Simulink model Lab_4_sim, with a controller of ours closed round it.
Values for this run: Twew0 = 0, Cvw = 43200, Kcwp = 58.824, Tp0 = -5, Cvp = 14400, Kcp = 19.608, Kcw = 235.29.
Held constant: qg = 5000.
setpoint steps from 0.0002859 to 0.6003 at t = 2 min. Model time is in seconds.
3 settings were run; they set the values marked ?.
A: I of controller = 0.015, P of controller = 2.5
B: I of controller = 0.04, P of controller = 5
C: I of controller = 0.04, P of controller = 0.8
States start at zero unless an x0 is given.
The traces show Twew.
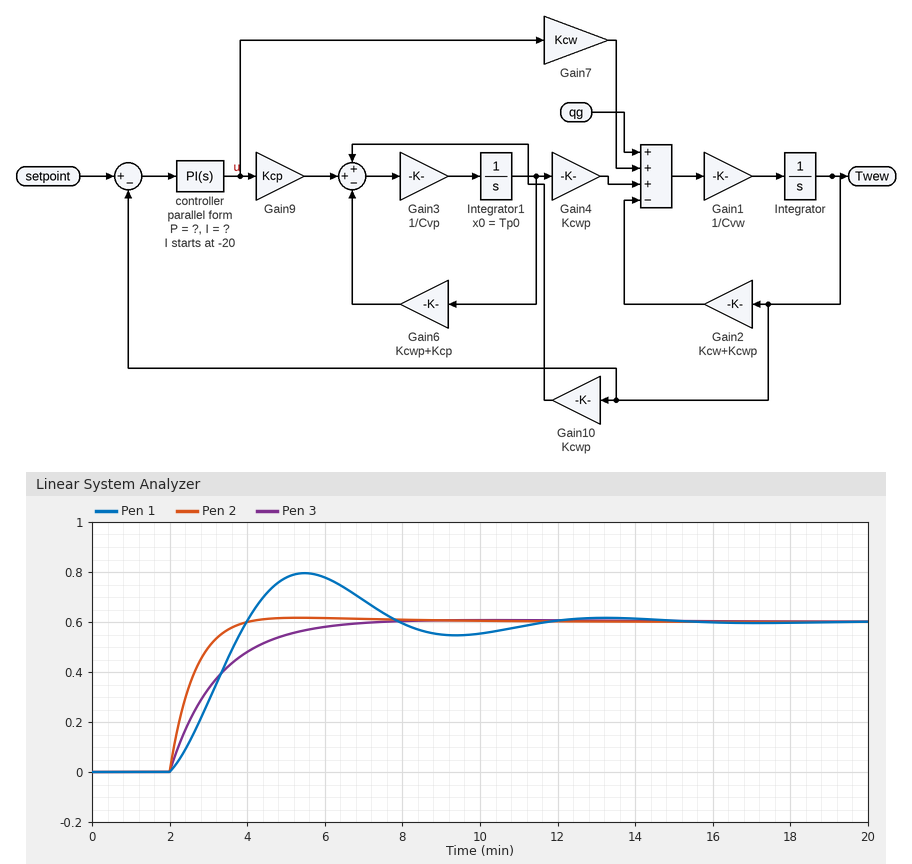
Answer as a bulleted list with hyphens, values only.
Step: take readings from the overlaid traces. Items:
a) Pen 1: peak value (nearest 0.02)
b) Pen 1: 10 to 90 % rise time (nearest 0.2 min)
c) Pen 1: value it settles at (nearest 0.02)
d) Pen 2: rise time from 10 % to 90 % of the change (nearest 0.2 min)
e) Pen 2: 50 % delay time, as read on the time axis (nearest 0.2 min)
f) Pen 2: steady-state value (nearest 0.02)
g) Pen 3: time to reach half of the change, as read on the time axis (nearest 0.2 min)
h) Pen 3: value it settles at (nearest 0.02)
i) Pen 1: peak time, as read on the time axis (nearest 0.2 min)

- 0.80
- 1.4 min
- 0.60
- 1.2 min
- 2.4 min
- 0.60
- 2.8 min
- 0.60
- 5.4 min
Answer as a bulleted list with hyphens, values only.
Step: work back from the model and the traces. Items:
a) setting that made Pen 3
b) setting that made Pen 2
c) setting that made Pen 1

- A
- B
- C
